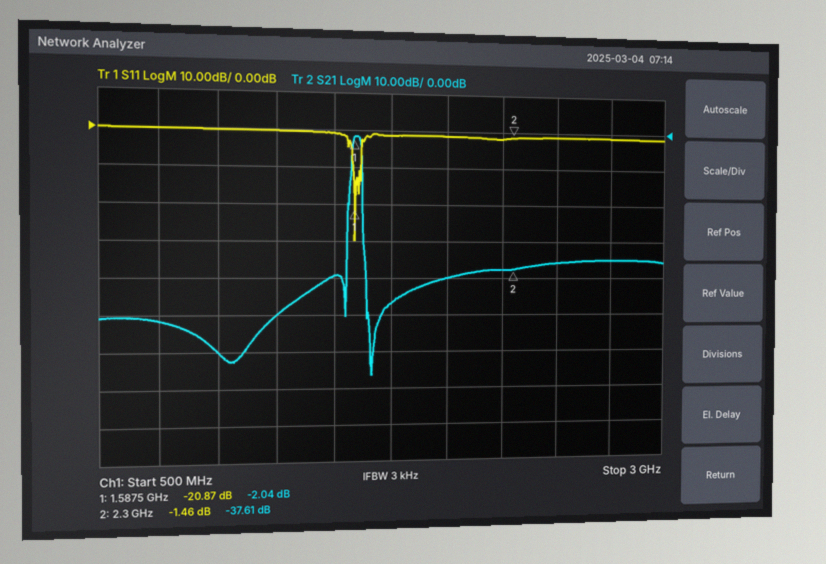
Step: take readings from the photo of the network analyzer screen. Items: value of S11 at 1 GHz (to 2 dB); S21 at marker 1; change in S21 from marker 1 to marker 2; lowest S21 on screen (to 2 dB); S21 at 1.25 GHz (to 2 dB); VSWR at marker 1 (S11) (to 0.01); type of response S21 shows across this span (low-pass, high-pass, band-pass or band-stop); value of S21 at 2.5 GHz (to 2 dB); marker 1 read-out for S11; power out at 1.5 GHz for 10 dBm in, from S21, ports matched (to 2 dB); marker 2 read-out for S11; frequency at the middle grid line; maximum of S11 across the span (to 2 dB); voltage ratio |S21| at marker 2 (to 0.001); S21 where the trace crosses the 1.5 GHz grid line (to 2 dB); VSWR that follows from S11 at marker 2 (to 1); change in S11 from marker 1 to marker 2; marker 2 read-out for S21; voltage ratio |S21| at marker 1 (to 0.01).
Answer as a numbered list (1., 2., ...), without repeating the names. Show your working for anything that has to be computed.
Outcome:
1. 0 dB
2. -2.04 dB
3. -37.61 − (-2.04) = -35.57 dB
4. -66 dB
5. -50 dB
6. (1 + 0.0905)/(1 − 0.0905) ≈ 1.20
7. band-pass
8. -36 dB
9. -20.87 dB
10. 10 dBm + (-40 dB) = -30 dBm
11. -1.46 dB
12. 1.75 GHz
13. 0 dB
14. 10^(-37.61/20) ≈ 0.013
15. -40 dB
16. (1 + 0.8453)/(1 − 0.8453) ≈ 12
17. -1.46 − (-20.87) = 19.41 dB
18. -37.61 dB
19. 10^(-2.04/20) ≈ 0.79
